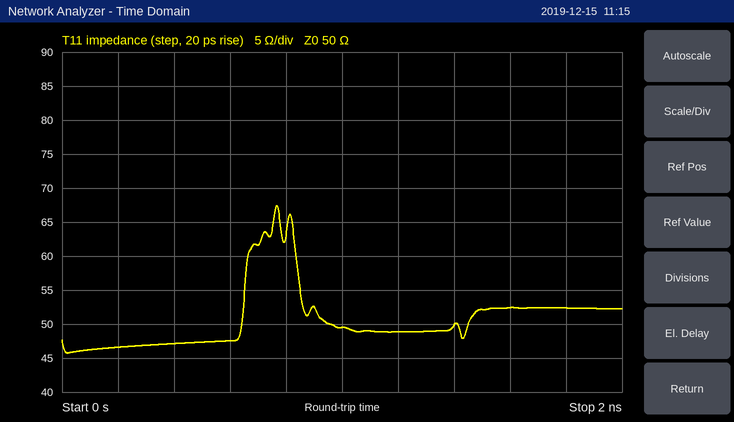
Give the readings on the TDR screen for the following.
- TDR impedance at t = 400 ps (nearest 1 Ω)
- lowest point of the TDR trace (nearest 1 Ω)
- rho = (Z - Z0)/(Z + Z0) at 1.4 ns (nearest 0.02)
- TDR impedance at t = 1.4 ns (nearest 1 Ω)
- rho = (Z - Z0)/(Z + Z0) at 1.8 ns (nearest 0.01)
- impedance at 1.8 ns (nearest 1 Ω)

47 Ω
46 Ω
0.00
50 Ω
+0.02
52 Ω
